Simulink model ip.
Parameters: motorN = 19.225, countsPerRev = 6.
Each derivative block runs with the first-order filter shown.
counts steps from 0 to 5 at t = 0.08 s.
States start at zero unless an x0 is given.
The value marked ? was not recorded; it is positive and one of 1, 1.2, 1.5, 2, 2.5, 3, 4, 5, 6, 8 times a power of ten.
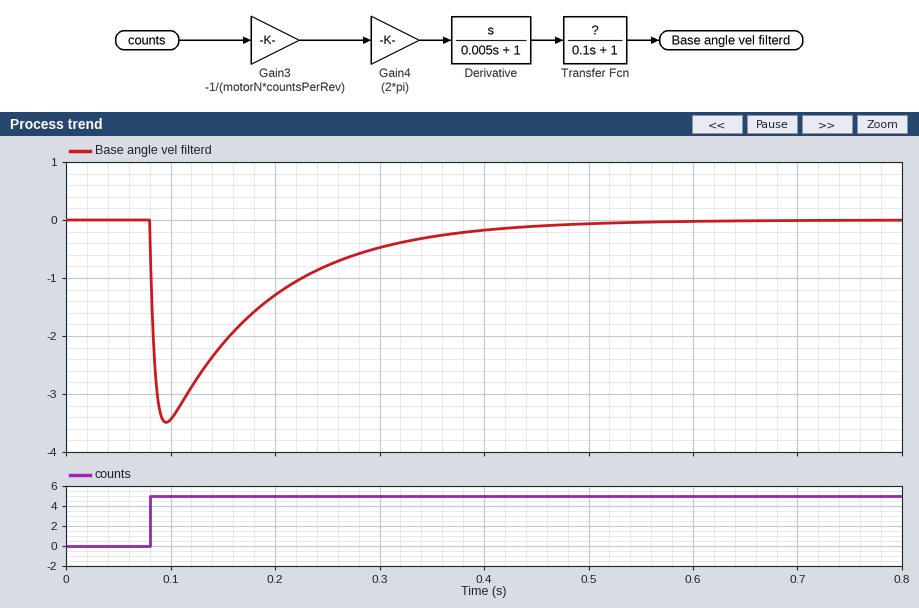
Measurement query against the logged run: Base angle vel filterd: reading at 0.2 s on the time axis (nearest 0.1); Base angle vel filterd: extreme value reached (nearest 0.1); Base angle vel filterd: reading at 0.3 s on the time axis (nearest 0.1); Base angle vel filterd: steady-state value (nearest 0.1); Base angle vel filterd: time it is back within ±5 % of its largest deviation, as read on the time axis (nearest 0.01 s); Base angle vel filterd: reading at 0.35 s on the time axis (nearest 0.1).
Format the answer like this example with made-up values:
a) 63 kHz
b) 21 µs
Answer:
a) -1.3
b) -3.5
c) -0.5
d) 0.0
e) 0.40 s
f) -0.3
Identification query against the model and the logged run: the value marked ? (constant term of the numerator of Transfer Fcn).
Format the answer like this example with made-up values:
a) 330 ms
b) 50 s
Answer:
a) 1.5
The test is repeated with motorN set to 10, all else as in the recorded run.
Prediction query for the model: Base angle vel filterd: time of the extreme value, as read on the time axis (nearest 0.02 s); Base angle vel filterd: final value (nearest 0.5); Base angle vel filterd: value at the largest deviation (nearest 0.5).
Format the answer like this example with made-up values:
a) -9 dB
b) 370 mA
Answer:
a) 0.10 s
b) 0.0
c) -6.5
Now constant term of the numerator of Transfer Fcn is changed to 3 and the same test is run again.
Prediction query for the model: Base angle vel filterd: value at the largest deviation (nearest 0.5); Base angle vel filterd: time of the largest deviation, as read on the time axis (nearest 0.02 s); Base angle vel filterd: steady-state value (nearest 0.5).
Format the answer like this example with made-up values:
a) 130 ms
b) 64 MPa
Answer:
a) -7.0
b) 0.10 s
c) 0.0
